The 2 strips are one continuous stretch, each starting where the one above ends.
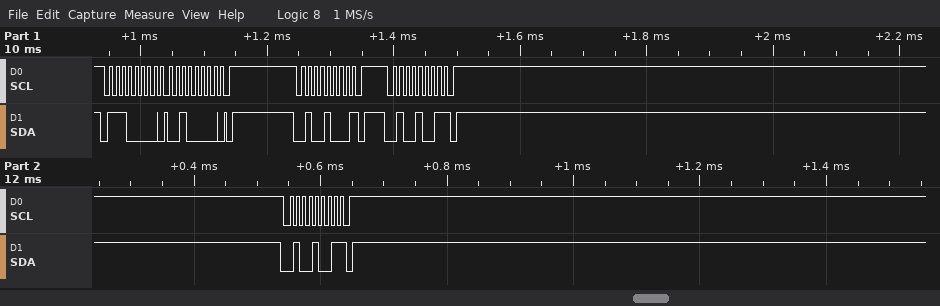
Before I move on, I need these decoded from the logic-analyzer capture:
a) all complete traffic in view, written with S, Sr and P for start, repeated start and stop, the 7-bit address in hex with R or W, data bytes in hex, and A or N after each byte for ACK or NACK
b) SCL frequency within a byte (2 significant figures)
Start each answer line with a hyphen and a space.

- S 70W A 20 A P S 24W N P S 24R N P S 24R N P
- 100 kHz
